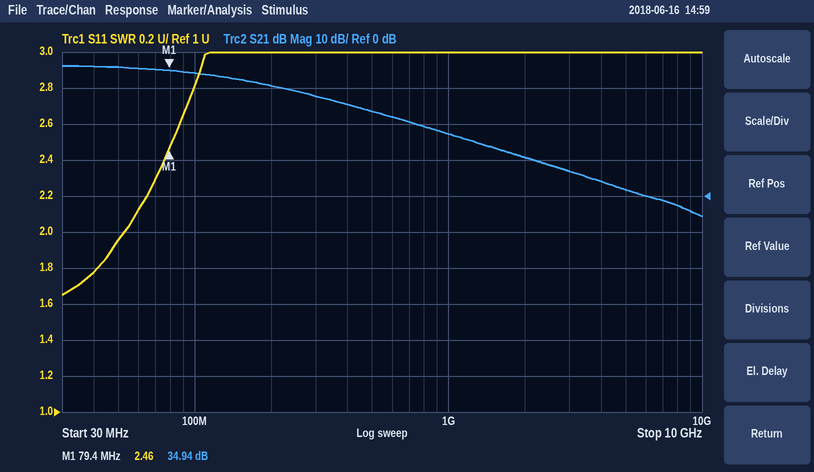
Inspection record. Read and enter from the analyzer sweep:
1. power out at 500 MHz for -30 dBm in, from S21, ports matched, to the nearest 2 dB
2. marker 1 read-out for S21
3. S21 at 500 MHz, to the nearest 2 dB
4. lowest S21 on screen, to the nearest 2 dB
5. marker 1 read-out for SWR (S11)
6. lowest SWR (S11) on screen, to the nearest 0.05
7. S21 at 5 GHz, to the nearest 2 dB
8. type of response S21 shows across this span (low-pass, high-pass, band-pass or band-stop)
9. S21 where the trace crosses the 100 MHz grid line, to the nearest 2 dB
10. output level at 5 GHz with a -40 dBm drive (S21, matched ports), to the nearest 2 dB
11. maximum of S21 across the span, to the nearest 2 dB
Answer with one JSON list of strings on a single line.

["-6 dBm", "34.94 dB", "24 dB", "-6 dB", "2.46", "1.65", "2 dB", "low-pass", "34 dB", "-38 dBm", "36 dB"]
